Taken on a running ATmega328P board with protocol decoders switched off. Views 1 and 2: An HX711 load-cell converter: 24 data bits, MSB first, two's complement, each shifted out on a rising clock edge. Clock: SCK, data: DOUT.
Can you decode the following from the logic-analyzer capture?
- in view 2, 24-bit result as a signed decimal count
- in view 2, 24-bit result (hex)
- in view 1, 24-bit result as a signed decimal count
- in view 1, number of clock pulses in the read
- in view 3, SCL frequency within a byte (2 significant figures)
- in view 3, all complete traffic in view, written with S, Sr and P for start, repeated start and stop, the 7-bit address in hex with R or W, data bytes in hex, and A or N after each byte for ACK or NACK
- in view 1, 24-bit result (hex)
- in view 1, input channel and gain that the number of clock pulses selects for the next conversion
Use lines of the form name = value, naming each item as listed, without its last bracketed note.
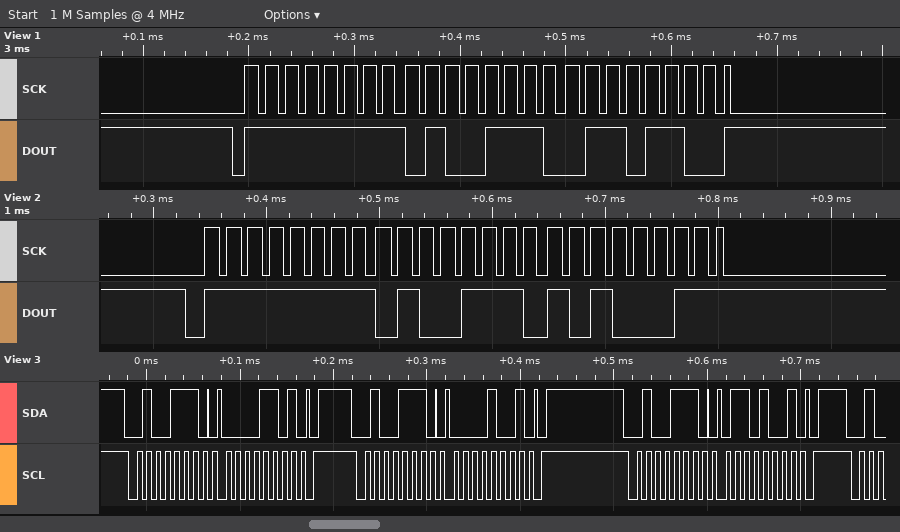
in view 2, 24-bit result as a signed decimal count = -45405
in view 2, 24-bit result = 0xFF4EA3
in view 1, 24-bit result as a signed decimal count = -45460
in view 1, number of clock pulses in the read = 25
in view 3, SCL frequency within a byte = 100 kHz
in view 3, all complete traffic in view, written with S, Sr and P for start, repeated start and stop, the 7-bit address in hex with R or W, data bytes in hex, and A or N after each byte for ACK or NACK = S 27W A 0D A P S 27W A 09 A P S 27W A 69 A P
in view 1, 24-bit result = 0xFF4E6C
in view 1, input channel and gain that the number of clock pulses selects for the next conversion = channel A, gain 128
